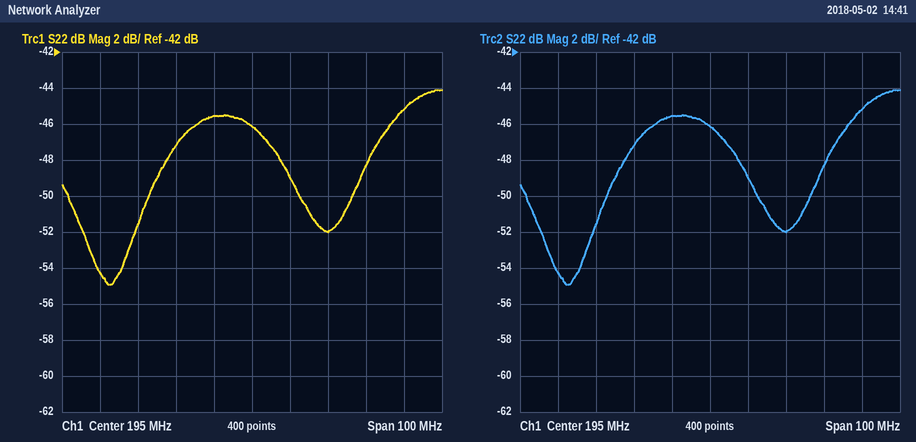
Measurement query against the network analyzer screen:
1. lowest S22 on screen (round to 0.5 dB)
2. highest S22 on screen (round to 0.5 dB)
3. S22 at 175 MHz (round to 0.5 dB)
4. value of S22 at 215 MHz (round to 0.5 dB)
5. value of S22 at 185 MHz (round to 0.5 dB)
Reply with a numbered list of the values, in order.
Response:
1. -55.0 dB
2. -44.0 dB
3. -47.0 dB
4. -52.0 dB
5. -45.5 dB
